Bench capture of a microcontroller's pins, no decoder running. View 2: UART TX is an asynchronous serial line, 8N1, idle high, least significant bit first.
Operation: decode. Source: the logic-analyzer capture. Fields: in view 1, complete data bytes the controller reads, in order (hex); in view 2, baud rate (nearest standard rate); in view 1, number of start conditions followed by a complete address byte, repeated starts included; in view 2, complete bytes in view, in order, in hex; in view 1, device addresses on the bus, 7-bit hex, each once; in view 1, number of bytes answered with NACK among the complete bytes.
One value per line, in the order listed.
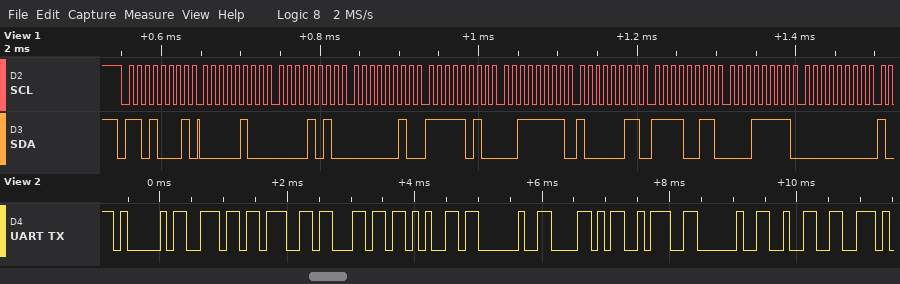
04 0A 02 FA 3F 83 F3 1F 00
9600 baud
1
41 6E 67 6C 65 20 58 3A 20 32
0x68
0
